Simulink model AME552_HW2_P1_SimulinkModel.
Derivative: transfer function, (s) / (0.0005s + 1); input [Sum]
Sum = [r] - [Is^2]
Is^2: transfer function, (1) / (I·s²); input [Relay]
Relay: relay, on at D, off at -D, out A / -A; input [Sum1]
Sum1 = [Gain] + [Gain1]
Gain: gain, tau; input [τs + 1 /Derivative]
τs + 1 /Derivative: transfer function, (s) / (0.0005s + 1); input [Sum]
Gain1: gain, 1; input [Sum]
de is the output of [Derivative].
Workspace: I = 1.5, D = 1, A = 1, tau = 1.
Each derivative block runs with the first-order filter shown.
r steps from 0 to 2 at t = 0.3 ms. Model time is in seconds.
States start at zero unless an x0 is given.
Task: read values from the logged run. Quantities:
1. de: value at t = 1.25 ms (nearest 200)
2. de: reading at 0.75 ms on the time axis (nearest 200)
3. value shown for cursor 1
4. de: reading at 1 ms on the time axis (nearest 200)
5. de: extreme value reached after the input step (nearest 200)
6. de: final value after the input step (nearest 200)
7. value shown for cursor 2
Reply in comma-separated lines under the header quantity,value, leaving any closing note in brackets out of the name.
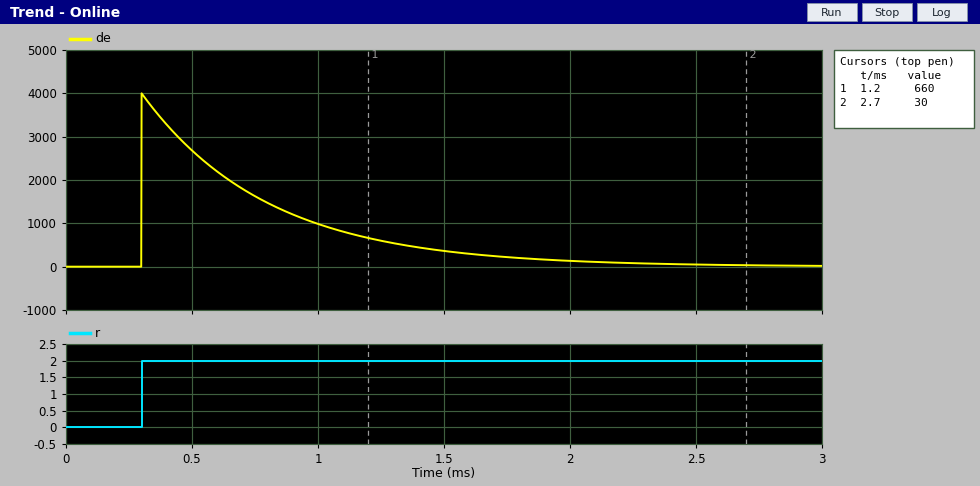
quantity,value
de: value at t = 1.25 ms,600
de: reading at 0.75 ms on the time axis,1600
value shown for cursor 1,660
de: reading at 1 ms on the time axis,1000
de: extreme value reached after the input step,4000
de: final value after the input step,0
value shown for cursor 2,30
